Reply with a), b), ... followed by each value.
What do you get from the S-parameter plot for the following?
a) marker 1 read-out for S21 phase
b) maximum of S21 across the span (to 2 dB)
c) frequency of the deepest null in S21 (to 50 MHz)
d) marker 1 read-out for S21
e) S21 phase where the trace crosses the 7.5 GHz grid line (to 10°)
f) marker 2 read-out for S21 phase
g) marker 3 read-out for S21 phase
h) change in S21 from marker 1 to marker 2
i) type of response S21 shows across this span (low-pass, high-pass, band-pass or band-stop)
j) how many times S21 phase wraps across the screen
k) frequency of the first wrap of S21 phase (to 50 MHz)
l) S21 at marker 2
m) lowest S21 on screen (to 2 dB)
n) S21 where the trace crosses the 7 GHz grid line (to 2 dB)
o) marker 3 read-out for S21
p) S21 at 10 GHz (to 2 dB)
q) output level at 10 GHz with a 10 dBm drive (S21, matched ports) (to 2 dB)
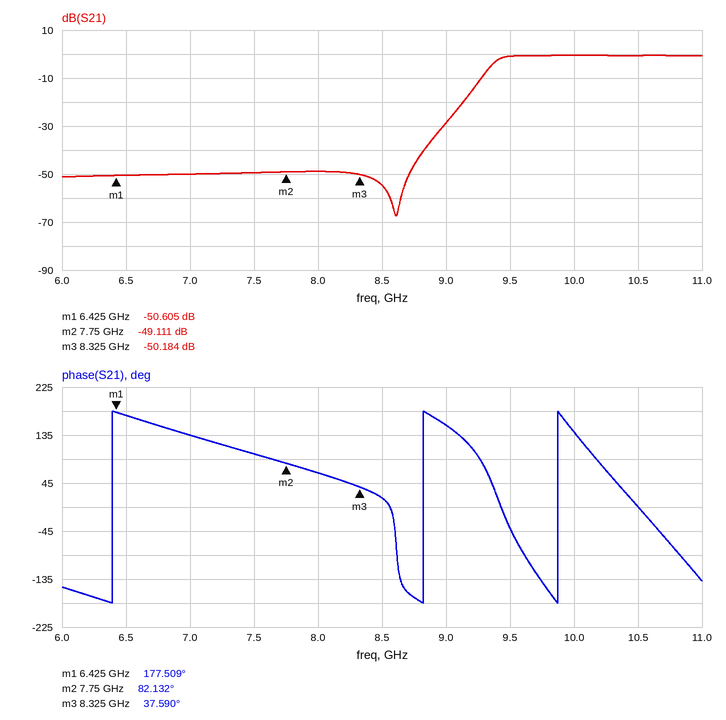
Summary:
a) 177.509°
b) 0 dB
c) 8.60 GHz
d) -50.605 dB
e) 100°
f) 82.132°
g) 37.590°
h) 1.494 dB
i) high-pass
j) 3
k) 6.40 GHz
l) -49.111 dB
m) -68 dB
n) -50 dB
o) -50.184 dB
p) 0 dB
q) 10 dBm
